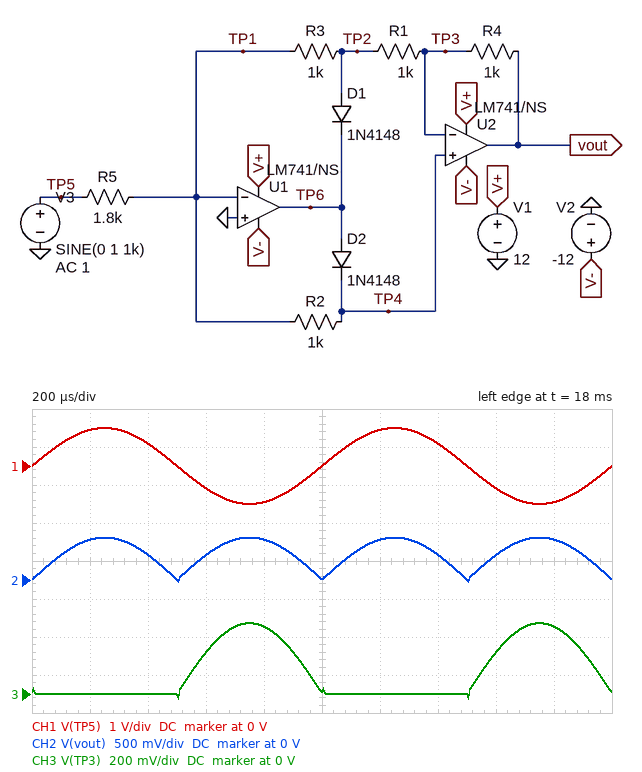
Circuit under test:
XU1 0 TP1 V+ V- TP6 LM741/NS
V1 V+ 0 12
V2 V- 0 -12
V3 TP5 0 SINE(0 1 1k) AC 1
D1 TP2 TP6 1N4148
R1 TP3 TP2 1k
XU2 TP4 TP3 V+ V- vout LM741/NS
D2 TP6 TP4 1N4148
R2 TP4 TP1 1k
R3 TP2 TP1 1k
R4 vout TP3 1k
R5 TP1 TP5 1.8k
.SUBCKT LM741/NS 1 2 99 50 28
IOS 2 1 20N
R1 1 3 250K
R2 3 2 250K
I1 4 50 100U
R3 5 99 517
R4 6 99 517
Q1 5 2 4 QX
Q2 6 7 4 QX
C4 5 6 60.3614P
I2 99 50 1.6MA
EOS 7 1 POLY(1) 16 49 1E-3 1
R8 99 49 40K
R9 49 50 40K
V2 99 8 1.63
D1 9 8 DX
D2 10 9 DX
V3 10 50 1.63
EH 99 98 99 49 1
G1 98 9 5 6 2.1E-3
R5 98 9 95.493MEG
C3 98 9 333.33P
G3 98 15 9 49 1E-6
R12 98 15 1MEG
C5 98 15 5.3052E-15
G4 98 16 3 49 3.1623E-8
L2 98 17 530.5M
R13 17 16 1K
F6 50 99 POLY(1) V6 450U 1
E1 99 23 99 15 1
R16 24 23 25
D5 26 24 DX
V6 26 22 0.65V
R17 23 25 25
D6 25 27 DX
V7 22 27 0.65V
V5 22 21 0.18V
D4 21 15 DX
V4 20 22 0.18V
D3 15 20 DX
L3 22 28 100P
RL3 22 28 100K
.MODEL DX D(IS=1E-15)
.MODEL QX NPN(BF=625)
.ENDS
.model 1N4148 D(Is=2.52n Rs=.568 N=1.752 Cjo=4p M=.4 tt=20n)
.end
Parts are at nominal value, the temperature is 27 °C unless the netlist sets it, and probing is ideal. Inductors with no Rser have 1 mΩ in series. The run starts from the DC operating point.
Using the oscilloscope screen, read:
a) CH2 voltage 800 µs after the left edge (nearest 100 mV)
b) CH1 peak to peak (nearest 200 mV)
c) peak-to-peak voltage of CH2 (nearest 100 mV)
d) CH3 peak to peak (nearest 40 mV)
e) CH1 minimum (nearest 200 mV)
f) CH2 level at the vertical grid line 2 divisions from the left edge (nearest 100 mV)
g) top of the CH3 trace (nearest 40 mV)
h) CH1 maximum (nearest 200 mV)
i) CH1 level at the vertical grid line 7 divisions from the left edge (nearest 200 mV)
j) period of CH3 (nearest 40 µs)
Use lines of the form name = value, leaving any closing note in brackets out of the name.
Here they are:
CH2 voltage 800 µs after the left edge = 500 mV
CH1 peak to peak = 2.0 V
peak-to-peak voltage of CH2 = 600 mV
CH3 peak to peak = 400 mV
CH1 minimum = -1.0 V
CH2 level at the vertical grid line 2 divisions from the left edge = 300 mV
top of the CH3 trace = 360 mV
CH1 maximum = 1.0 V
CH1 level at the vertical grid line 7 divisions from the left edge = 600 mV
period of CH3 = 1.00 ms
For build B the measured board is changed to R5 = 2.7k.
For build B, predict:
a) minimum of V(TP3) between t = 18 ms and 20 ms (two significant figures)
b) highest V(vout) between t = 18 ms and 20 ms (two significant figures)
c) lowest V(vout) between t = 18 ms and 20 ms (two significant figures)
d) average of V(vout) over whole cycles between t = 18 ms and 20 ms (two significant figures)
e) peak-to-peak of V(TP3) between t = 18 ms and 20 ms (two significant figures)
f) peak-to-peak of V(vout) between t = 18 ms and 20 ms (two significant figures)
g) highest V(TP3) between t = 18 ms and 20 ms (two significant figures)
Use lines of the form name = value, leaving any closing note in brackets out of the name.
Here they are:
minimum of V(TP3) between t = 18 ms and 20 ms = -27 mV
highest V(vout) between t = 18 ms and 20 ms = 370 mV
lowest V(vout) between t = 18 ms and 20 ms = -26 mV
average of V(vout) over whole cycles between t = 18 ms and 20 ms = 240 mV
peak-to-peak of V(TP3) between t = 18 ms and 20 ms = 280 mV
peak-to-peak of V(vout) between t = 18 ms and 20 ms = 400 mV
highest V(TP3) between t = 18 ms and 20 ms = 250 mV
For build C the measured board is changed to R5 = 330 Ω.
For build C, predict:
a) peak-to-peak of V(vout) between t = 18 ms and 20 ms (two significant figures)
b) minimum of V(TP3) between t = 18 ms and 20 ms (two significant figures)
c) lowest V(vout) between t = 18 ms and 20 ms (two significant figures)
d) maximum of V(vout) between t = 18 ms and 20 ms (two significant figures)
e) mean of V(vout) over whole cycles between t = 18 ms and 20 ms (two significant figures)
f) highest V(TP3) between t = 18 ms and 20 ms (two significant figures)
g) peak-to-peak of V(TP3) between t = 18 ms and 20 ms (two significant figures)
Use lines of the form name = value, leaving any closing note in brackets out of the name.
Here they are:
peak-to-peak of V(vout) between t = 18 ms and 20 ms = 3.1 V
minimum of V(TP3) between t = 18 ms and 20 ms = -34 mV
lowest V(vout) between t = 18 ms and 20 ms = -33 mV
maximum of V(vout) between t = 18 ms and 20 ms = 3.0 V
mean of V(vout) over whole cycles between t = 18 ms and 20 ms = 1.9 V
highest V(TP3) between t = 18 ms and 20 ms = 2.0 V
peak-to-peak of V(TP3) between t = 18 ms and 20 ms = 2.1 V
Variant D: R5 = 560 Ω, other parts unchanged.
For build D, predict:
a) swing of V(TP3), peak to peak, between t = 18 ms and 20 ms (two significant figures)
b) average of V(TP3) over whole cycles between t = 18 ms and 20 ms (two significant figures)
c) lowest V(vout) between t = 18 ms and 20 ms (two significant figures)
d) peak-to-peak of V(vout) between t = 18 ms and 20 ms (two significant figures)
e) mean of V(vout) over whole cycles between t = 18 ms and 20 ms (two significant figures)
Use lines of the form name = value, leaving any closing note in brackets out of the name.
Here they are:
swing of V(TP3), peak to peak, between t = 18 ms and 20 ms = 1.2 V
average of V(TP3) over whole cycles between t = 18 ms and 20 ms = 380 mV
lowest V(vout) between t = 18 ms and 20 ms = -31 mV
peak-to-peak of V(vout) between t = 18 ms and 20 ms = 1.8 V
mean of V(vout) over whole cycles between t = 18 ms and 20 ms = 1.1 V
